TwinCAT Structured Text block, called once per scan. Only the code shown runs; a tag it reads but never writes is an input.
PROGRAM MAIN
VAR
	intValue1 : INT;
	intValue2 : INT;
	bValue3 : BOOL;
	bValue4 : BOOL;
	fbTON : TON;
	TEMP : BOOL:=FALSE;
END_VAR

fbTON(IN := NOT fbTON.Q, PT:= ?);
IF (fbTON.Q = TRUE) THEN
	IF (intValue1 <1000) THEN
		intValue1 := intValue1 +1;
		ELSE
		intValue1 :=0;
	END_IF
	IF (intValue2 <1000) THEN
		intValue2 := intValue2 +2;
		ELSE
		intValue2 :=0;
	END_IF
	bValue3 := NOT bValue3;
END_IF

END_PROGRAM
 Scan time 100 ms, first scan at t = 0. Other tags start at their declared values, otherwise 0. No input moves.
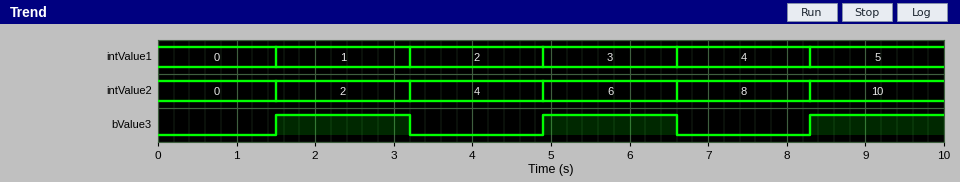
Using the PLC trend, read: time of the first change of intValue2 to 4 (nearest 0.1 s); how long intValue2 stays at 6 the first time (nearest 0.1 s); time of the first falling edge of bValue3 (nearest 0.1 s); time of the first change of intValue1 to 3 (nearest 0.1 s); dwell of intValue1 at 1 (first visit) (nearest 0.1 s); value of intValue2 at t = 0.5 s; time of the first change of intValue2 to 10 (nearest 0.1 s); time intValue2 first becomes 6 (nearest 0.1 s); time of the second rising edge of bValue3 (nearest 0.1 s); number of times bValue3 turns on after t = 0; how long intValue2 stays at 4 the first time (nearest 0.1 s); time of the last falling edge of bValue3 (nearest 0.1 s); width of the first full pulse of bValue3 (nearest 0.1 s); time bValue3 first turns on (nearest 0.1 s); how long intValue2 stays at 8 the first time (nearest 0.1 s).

3.2 s
1.7 s
3.2 s
4.9 s
1.7 s
0
8.3 s
4.9 s
4.9 s
3
1.7 s
6.6 s
1.7 s
1.5 s
1.7 s
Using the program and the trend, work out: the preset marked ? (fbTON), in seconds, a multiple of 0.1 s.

1.5 s
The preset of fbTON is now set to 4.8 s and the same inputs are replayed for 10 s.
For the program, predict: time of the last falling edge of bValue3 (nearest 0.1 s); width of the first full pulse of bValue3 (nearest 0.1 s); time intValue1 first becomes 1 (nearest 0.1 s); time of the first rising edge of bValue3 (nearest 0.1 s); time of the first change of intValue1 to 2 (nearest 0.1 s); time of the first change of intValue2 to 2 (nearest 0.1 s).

9.8 s
5.0 s
4.8 s
4.8 s
9.8 s
4.8 s
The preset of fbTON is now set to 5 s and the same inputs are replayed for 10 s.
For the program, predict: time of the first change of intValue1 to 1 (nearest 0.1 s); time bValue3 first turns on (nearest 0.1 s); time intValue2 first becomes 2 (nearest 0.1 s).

5.0 s
5.0 s
5.0 s
